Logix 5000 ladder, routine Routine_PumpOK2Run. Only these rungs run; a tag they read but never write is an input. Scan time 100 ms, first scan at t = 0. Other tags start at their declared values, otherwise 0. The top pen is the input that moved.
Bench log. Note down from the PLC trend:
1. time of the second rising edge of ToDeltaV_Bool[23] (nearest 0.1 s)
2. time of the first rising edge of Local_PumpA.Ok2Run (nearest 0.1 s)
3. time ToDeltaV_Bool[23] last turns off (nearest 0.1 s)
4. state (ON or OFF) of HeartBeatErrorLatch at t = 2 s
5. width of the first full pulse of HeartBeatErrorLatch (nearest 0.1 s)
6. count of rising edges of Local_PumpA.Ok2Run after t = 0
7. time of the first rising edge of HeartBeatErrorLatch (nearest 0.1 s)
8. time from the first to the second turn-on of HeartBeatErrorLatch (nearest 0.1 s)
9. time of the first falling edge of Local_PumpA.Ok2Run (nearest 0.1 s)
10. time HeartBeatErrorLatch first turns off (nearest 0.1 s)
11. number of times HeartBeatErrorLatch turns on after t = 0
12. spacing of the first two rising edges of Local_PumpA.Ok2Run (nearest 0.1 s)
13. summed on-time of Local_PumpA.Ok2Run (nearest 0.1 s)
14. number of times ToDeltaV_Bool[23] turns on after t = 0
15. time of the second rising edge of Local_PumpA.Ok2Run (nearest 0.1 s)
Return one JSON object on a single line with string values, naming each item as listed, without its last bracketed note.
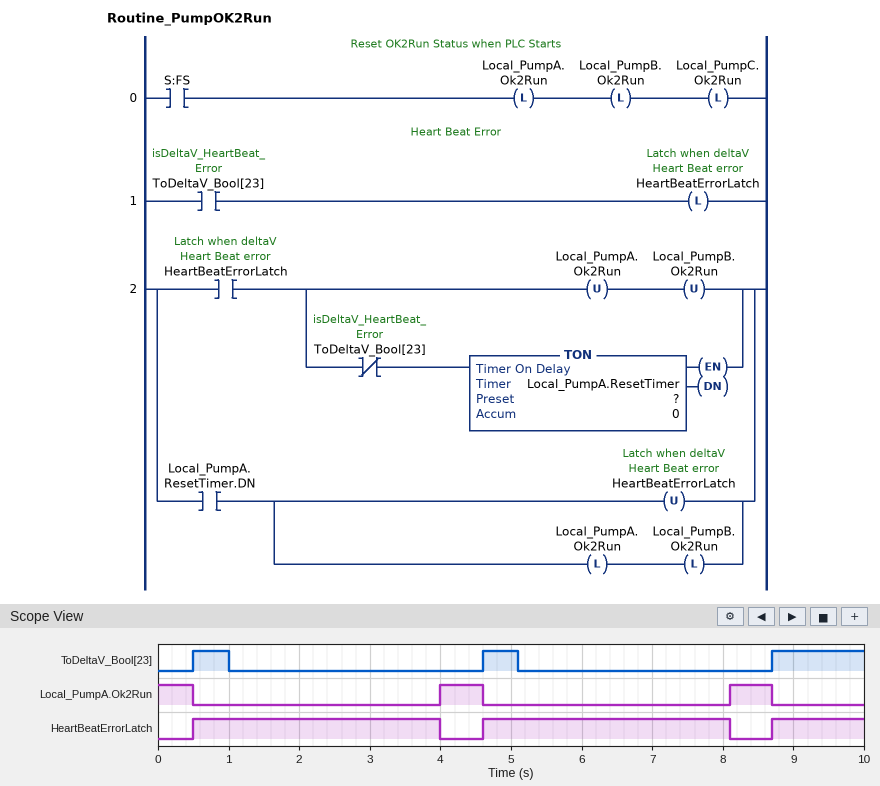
{"time of the second rising edge of ToDeltaV_Bool[23]": "4.6 s", "time of the first rising edge of Local_PumpA.Ok2Run": "4.0 s", "time ToDeltaV_Bool[23] last turns off": "5.1 s", "state (ON or OFF) of HeartBeatErrorLatch at t = 2 s": "ON", "width of the first full pulse of HeartBeatErrorLatch": "3.5 s", "count of rising edges of Local_PumpA.Ok2Run after t = 0": "2", "time of the first rising edge of HeartBeatErrorLatch": "0.5 s", "time from the first to the second turn-on of HeartBeatErrorLatch": "4.1 s", "time of the first falling edge of Local_PumpA.Ok2Run": "0.5 s", "time HeartBeatErrorLatch first turns off": "4.0 s", "number of times HeartBeatErrorLatch turns on after t = 0": "3", "spacing of the first two rising edges of Local_PumpA.Ok2Run": "4.1 s", "summed on-time of Local_PumpA.Ok2Run": "1.7 s", "number of times ToDeltaV_Bool[23] turns on after t = 0": "3", "time of the second rising edge of Local_PumpA.Ok2Run": "8.1 s"}
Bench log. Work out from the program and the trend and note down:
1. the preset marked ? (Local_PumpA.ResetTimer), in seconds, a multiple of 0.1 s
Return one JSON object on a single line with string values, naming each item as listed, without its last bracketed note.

{"the preset marked ? (Local_PumpA.ResetTimer), in seconds, a multiple of 0.1 s": "3.0 s"}
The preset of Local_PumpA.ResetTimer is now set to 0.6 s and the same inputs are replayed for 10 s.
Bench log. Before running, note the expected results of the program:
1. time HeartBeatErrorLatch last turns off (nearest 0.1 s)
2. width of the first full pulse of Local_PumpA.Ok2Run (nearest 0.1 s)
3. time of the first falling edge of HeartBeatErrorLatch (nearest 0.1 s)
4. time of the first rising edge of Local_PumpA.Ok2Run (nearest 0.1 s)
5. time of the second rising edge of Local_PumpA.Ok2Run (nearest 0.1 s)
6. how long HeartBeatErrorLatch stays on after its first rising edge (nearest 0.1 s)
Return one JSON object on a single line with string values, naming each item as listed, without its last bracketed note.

{"time HeartBeatErrorLatch last turns off": "5.7 s", "width of the first full pulse of Local_PumpA.Ok2Run": "3.0 s", "time of the first falling edge of HeartBeatErrorLatch": "1.6 s", "time of the first rising edge of Local_PumpA.Ok2Run": "1.6 s", "time of the second rising edge of Local_PumpA.Ok2Run": "5.7 s", "how long HeartBeatErrorLatch stays on after its first rising edge": "1.1 s"}
